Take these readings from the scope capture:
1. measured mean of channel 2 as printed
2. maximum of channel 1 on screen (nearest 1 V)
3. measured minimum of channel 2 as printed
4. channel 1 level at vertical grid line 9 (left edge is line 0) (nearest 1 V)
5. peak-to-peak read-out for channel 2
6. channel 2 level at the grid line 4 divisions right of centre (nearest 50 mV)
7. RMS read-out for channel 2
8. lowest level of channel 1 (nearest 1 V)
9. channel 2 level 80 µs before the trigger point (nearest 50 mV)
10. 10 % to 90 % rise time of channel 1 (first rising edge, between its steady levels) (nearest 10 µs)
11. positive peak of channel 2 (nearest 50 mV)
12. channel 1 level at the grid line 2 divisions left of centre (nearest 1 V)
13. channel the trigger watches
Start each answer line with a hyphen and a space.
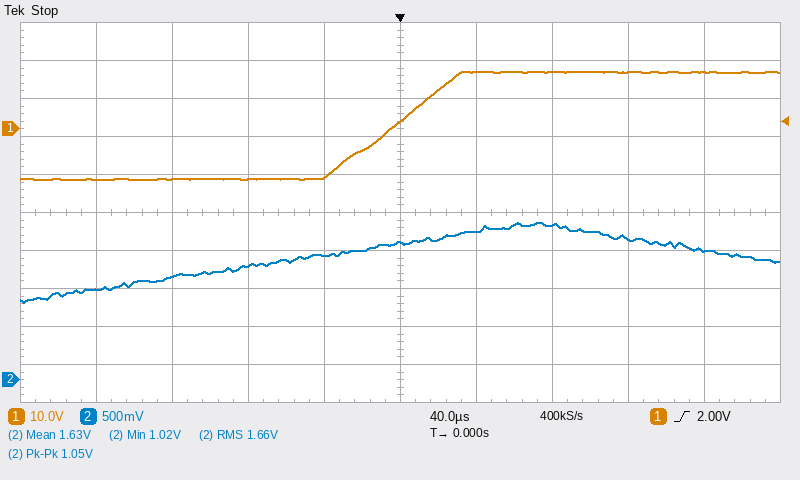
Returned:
- 1.63 V
- 15 V
- 1.02 V
- 15 V
- 1.05 V
- 1.70 V
- 1.66 V
- -13 V
- 1.50 V
- 60 µs
- 2.05 V
- -13 V
- channel 1
